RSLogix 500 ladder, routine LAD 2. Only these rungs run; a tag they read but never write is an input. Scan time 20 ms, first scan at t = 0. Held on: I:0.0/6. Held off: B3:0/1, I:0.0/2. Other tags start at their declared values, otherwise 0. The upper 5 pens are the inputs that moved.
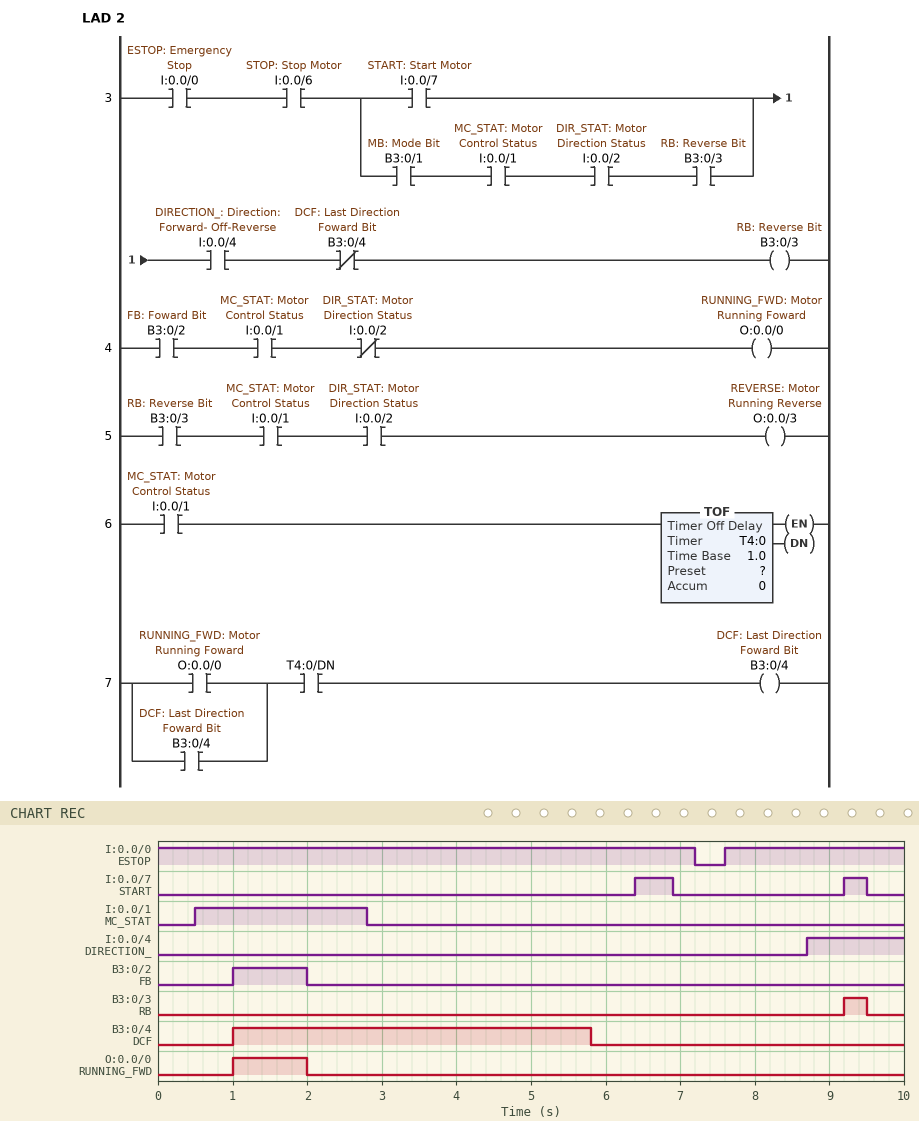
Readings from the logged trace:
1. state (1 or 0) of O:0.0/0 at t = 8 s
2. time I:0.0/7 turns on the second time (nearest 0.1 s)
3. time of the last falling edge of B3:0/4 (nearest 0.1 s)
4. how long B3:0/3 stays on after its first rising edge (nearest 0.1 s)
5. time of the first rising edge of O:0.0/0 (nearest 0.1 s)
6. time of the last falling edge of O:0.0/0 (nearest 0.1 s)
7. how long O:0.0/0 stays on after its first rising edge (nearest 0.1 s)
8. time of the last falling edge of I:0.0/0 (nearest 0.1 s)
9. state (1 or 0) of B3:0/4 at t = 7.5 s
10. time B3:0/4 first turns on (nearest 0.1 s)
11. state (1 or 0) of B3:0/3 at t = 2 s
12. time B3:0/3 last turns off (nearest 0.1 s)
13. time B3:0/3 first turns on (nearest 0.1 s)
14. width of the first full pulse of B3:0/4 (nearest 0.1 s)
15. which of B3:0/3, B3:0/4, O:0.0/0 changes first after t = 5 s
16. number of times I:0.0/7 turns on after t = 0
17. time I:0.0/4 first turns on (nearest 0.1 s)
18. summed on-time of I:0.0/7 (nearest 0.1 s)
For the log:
0
9.2 s
5.8 s
0.3 s
1.0 s
2.0 s
1.0 s
7.2 s
0
1.0 s
0
9.5 s
9.2 s
4.8 s
B3:0/4
2
8.7 s
0.8 s
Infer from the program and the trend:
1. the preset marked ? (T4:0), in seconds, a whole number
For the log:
3 s
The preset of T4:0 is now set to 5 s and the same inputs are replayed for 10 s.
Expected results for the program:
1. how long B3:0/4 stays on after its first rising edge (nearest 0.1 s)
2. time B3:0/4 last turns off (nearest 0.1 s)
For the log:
6.8 s
7.8 s
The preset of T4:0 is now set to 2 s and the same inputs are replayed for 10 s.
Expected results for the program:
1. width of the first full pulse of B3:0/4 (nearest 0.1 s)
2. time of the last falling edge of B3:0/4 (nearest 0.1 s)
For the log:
3.8 s
4.8 s
